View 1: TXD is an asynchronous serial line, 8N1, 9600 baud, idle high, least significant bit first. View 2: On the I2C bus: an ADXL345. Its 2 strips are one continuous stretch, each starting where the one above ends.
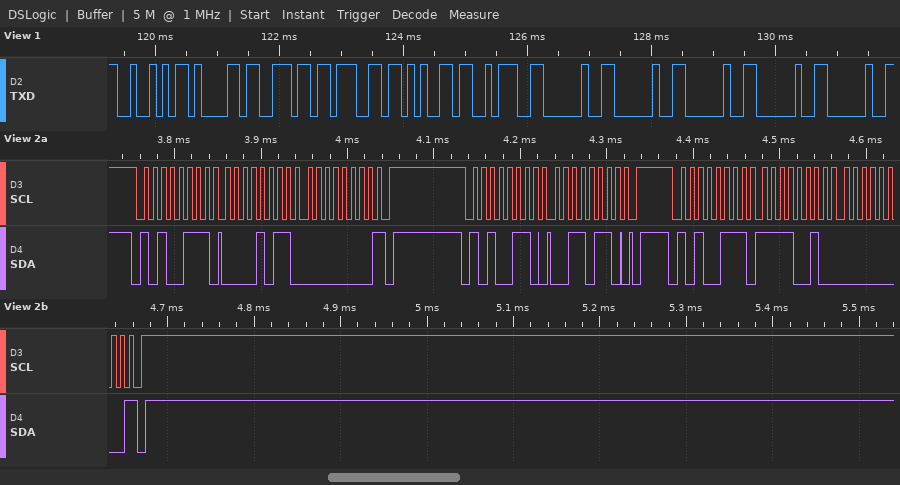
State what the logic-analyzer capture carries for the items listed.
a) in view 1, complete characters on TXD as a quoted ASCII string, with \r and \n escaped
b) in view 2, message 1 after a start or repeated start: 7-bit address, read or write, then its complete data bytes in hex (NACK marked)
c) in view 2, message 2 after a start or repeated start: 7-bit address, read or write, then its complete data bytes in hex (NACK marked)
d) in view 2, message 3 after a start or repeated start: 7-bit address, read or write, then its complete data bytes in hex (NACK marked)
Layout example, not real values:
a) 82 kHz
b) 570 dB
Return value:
a) "Range:     "
b) 0x53 read: 0B 00 NACK
c) 0x53 write: 36
d) 0x53 read: F2 00 NACK
